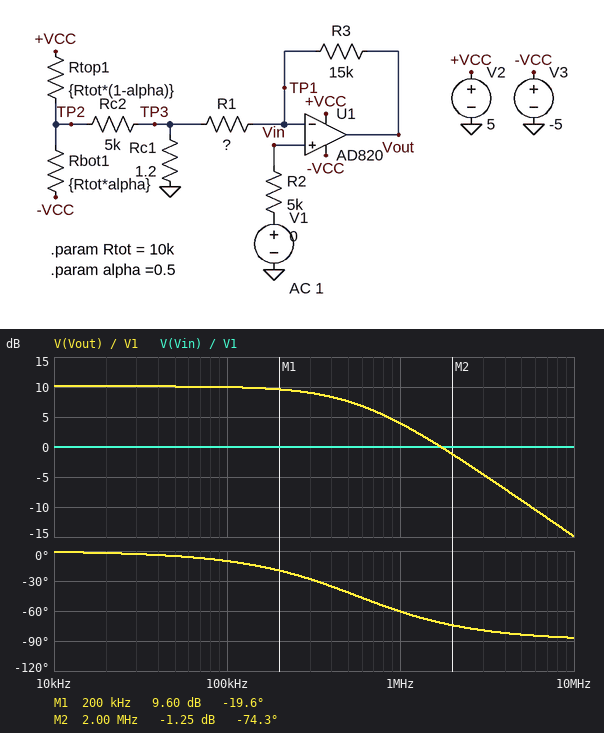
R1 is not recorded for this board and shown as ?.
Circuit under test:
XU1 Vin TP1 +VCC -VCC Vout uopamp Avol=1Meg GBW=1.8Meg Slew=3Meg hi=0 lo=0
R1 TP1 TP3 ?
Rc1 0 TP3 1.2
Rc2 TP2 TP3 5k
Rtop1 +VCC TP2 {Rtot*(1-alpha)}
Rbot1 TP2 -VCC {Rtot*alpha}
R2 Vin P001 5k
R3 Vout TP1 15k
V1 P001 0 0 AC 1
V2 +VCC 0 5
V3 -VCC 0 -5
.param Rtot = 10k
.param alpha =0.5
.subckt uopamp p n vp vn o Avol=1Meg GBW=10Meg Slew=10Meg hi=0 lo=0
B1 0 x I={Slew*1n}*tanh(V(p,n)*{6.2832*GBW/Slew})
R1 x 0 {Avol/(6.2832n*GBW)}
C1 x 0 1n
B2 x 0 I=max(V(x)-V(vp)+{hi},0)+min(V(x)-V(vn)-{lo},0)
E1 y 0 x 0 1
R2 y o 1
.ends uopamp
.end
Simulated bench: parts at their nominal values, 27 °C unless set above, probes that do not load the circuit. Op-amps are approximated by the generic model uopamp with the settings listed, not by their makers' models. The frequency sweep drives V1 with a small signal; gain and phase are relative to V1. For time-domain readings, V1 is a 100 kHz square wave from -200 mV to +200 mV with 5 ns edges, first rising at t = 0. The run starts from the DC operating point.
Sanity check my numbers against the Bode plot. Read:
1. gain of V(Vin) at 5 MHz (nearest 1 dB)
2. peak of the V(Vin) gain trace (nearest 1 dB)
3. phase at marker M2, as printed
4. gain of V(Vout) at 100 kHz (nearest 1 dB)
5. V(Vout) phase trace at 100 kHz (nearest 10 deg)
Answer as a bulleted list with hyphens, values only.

- 0 dB
- 0 dB
- -74.3 deg
- 10 dB
- -10 deg
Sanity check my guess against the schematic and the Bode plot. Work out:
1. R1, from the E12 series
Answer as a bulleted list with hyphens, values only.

- 6.8 kΩ
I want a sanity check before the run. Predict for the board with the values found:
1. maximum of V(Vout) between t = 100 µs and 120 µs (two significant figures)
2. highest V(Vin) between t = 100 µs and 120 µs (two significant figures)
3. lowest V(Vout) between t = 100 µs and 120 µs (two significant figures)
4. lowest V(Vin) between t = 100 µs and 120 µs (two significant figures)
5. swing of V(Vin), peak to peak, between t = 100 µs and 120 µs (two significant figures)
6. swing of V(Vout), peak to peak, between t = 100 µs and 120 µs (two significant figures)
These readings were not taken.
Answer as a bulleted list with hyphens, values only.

- 640 mV
- 200 mV
- -640 mV
- -200 mV
- 400 mV
- 1.3 V
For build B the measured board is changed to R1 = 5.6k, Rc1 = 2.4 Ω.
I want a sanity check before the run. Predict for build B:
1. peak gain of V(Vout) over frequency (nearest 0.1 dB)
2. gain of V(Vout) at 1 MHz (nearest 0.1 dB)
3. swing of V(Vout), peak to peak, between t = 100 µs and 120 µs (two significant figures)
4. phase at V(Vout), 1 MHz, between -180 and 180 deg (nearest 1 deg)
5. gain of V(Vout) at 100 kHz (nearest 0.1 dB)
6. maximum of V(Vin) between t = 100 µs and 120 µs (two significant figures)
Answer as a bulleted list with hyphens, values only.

- 11.3 dB
- 4.2 dB
- 1.5 V
- -64 deg
- 11.1 dB
- 200 mV
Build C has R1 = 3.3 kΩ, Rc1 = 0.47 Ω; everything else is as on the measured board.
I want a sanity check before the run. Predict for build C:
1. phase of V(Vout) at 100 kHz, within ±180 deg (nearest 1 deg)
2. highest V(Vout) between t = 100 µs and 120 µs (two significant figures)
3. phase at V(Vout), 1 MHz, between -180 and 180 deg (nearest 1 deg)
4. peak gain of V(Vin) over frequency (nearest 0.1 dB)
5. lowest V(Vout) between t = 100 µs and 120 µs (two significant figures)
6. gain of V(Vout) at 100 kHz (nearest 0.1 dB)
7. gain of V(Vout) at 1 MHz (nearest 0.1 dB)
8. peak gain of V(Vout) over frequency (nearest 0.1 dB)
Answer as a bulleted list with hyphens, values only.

- -17 deg
- 1.1 V
- -72 deg
- 0 dB
- -1.1 V
- 14.5 dB
- 4.7 dB
- 14.9 dB
